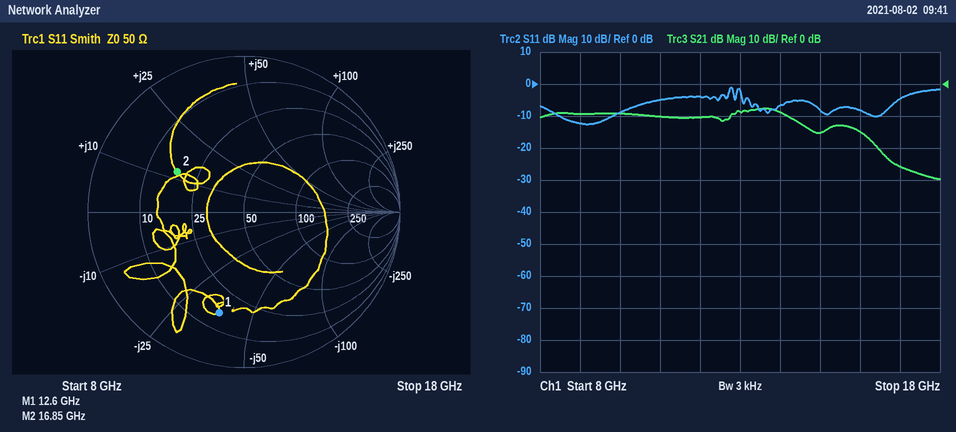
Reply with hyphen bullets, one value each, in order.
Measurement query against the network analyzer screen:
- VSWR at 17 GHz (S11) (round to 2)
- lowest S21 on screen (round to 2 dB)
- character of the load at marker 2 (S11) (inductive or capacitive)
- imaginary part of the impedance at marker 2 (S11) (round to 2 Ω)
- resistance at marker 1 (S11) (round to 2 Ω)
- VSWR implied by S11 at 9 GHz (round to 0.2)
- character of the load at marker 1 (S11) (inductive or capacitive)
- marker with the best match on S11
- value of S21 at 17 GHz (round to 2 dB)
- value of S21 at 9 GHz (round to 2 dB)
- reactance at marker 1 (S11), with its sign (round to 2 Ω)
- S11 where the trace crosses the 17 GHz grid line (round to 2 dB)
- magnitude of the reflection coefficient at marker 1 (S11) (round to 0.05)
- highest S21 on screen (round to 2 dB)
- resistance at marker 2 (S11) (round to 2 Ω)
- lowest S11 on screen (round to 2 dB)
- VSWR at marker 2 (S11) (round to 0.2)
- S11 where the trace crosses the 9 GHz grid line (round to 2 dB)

- 4
- -30 dB
- inductive
- +12 Ω
- 16 Ω
- 1.6
- capacitive
- marker 2
- -26 dB
- -10 dB
- -36 Ω
- -4 dB
- 0.65
- -8 dB
- 18 Ω
- -12 dB
- 3.0
- -12 dB
